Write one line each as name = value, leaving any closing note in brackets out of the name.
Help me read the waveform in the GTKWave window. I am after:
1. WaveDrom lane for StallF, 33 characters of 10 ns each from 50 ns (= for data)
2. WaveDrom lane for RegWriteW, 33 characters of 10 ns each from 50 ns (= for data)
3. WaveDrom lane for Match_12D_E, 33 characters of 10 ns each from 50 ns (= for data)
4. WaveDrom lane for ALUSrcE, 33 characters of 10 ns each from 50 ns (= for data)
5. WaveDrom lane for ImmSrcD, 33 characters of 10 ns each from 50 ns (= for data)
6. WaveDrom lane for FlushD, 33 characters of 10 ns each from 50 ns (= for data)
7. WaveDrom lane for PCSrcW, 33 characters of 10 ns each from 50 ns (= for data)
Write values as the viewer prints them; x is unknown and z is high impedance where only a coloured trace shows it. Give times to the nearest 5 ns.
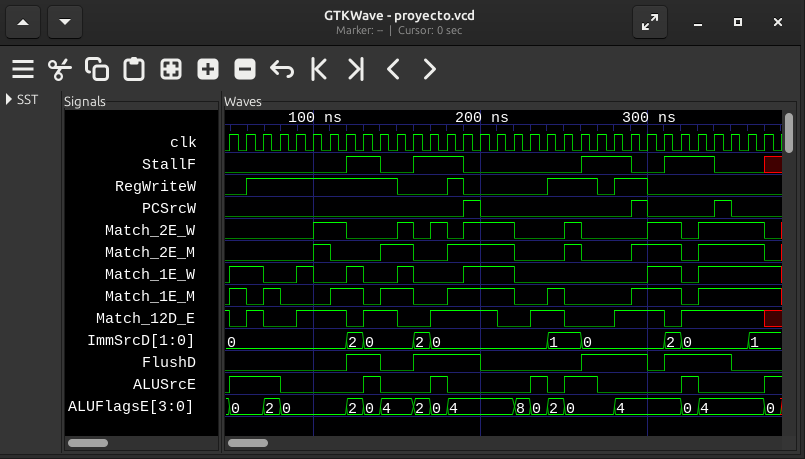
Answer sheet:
WaveDrom lane for StallF, 33 characters of 10 ns each from 50 ns = {name: 'StallF', wave: '0......1.0.1..0......1..0.1..0..x'}
WaveDrom lane for RegWriteW, 33 characters of 10 ns each from 50 ns = {name: 'RegWriteW', wave: '01........0..10....1..01.0.......'}
WaveDrom lane for Match_12D_E, 33 characters of 10 ns each from 50 ns = {name: 'Match_12D_E', wave: '010.1..01.0.1...0.1.0..1..01....x'}
WaveDrom lane for ALUSrcE, 33 characters of 10 ns each from 50 ns = {name: 'ALUSrcE', wave: '1..0....10..10....101.0....10...1'}
WaveDrom lane for ImmSrcD, 33 characters of 10 ns each from 50 ns = {name: 'ImmSrcD', wave: '=......==..==......=.=....==...=.', data: '0 2 0 2 0 1 0 2 0 1'}
WaveDrom lane for FlushD, 33 characters of 10 ns each from 50 ns = {name: 'FlushD', wave: '0......1.0.1...0.....1...01...0..'}
WaveDrom lane for PCSrcW, 33 characters of 10 ns each from 50 ns = {name: 'PCSrcW', wave: '0.............10........10...10..'}
